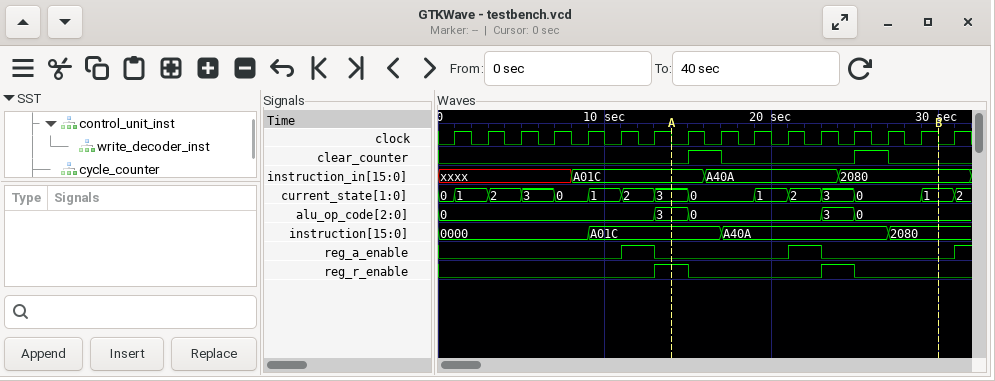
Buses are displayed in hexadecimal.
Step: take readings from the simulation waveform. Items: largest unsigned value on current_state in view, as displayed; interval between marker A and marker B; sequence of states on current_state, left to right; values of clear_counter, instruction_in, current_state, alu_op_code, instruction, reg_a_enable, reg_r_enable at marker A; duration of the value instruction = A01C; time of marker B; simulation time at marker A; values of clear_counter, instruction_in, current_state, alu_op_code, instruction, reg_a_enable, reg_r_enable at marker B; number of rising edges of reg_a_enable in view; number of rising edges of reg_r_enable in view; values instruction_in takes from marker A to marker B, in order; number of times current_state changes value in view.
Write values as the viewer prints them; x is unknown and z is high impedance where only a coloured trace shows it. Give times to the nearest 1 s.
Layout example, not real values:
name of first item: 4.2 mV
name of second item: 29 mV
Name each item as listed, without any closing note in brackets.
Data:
largest unsigned value on current_state in view, as displayed: 3
interval between marker A and marker B: 16 s
sequence of states on current_state, left to right: 0, 1, 2, 3, 0, 1, 2, 3, 0, 1, 2, 3, 0, 1, 2
values of clear_counter, instruction_in, current_state, alu_op_code, instruction, reg_a_enable, reg_r_enable at marker A: clear_counter=0, instruction_in=A01C, current_state=3, alu_op_code=3, instruction=A01C, reg_a_enable=0, reg_r_enable=1
duration of the value instruction = A01C: 8 s
time of marker B: 30 s
simulation time at marker A: 14 s
values of clear_counter, instruction_in, current_state, alu_op_code, instruction, reg_a_enable, reg_r_enable at marker B: clear_counter=0, instruction_in=2080, current_state=1, alu_op_code=0, instruction=2080, reg_a_enable=0, reg_r_enable=0
number of rising edges of reg_a_enable in view: 3
number of rising edges of reg_r_enable in view: 2
values instruction_in takes from marker A to marker B, in order: A01C, A40A, 2080
number of times current_state changes value in view: 14
